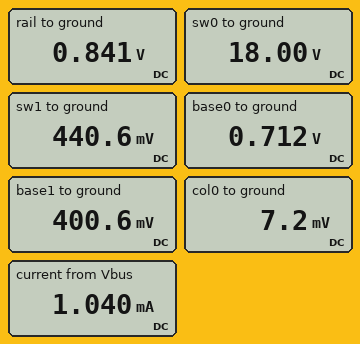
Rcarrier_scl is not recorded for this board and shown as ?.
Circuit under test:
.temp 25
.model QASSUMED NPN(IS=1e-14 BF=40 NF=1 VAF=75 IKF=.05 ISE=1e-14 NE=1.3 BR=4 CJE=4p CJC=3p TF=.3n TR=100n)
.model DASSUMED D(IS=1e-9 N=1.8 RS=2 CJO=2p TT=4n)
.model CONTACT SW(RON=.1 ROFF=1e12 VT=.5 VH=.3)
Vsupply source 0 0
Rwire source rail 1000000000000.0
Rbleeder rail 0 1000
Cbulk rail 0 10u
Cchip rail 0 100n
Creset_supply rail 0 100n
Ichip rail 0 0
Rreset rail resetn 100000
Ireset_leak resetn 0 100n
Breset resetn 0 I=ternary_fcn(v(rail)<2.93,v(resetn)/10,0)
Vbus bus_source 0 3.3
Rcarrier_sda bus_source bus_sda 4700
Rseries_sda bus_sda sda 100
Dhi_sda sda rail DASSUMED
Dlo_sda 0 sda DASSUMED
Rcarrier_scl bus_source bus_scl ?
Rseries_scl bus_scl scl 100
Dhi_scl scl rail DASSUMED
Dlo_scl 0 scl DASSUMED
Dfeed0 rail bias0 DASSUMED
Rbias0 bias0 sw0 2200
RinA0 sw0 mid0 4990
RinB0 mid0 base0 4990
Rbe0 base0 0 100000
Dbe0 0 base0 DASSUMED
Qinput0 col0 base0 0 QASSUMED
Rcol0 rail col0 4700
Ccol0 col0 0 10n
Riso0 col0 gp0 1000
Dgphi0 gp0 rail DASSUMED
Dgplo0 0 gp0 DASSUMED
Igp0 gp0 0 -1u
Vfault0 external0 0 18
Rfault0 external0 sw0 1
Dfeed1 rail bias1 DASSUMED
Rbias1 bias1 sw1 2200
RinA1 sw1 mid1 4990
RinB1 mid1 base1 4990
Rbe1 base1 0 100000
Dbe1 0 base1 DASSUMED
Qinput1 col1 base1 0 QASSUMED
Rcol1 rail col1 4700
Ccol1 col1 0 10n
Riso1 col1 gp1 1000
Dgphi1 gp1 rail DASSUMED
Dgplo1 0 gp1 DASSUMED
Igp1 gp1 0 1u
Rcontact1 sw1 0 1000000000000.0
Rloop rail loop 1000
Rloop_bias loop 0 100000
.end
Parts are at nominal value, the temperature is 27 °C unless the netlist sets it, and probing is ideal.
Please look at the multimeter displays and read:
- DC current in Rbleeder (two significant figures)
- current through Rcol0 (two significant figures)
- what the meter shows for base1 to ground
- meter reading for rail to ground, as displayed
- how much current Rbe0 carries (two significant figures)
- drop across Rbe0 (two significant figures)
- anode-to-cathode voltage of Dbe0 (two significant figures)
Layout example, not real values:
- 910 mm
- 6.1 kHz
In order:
- 840 µA
- 180 µA
- 400.6 mV
- 0.841 V
- 7.1 µA
- 710 mV
- -710 mV
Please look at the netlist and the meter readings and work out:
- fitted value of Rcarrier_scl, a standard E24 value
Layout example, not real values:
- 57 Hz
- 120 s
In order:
- 2.7 kΩ
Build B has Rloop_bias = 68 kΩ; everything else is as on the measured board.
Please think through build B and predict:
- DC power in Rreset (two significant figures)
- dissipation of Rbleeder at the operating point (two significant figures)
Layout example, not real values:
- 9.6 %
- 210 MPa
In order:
- 7.0 µW
- 700 µW
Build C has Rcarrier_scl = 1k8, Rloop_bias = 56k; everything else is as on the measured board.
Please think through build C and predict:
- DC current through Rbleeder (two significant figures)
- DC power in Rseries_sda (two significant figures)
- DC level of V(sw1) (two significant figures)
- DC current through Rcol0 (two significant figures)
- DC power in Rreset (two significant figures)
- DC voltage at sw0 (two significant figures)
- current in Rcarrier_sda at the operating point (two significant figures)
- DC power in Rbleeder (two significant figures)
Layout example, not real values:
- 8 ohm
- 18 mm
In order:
- 990 µA
- 13 µW
- 570 mV
- 210 µA
- 9.8 µW
- 18 V
- 360 µA
- 980 µW
